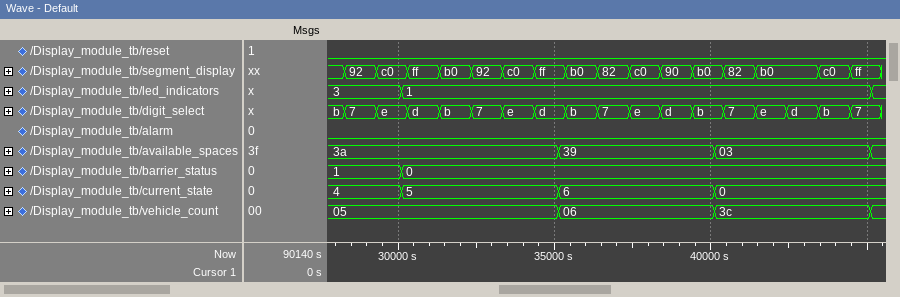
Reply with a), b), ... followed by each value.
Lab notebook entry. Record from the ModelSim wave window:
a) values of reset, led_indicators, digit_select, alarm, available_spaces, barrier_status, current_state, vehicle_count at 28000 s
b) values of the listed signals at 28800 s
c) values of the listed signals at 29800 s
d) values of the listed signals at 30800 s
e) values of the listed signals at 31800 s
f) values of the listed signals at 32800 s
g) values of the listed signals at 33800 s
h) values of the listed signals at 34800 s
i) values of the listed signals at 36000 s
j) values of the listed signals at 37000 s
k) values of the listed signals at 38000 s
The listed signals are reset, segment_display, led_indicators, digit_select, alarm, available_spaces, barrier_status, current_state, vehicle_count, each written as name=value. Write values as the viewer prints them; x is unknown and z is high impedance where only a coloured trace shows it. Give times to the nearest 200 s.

a) reset=0, led_indicators=3, digit_select=b, alarm=0, available_spaces=3a, barrier_status=1, current_state=4, vehicle_count=05
b) reset=0, segment_display=92, led_indicators=3, digit_select=7, alarm=0, available_spaces=3a, barrier_status=1, current_state=4, vehicle_count=05
c) reset=0, segment_display=c0, led_indicators=3, digit_select=e, alarm=0, available_spaces=3a, barrier_status=1, current_state=4, vehicle_count=05
d) reset=0, segment_display=ff, led_indicators=1, digit_select=d, alarm=0, available_spaces=3a, barrier_status=0, current_state=5, vehicle_count=05
e) reset=0, segment_display=b0, led_indicators=1, digit_select=b, alarm=0, available_spaces=3a, barrier_status=0, current_state=5, vehicle_count=05
f) reset=0, segment_display=92, led_indicators=1, digit_select=7, alarm=0, available_spaces=3a, barrier_status=0, current_state=5, vehicle_count=05
g) reset=0, segment_display=c0, led_indicators=1, digit_select=e, alarm=0, available_spaces=3a, barrier_status=0, current_state=5, vehicle_count=05
h) reset=0, segment_display=ff, led_indicators=1, digit_select=d, alarm=0, available_spaces=3a, barrier_status=0, current_state=5, vehicle_count=05
i) reset=0, segment_display=b0, led_indicators=1, digit_select=b, alarm=0, available_spaces=39, barrier_status=0, current_state=6, vehicle_count=06
j) reset=0, segment_display=82, led_indicators=1, digit_select=7, alarm=0, available_spaces=39, barrier_status=0, current_state=6, vehicle_count=06
k) reset=0, segment_display=c0, led_indicators=1, digit_select=e, alarm=0, available_spaces=39, barrier_status=0, current_state=6, vehicle_count=06
